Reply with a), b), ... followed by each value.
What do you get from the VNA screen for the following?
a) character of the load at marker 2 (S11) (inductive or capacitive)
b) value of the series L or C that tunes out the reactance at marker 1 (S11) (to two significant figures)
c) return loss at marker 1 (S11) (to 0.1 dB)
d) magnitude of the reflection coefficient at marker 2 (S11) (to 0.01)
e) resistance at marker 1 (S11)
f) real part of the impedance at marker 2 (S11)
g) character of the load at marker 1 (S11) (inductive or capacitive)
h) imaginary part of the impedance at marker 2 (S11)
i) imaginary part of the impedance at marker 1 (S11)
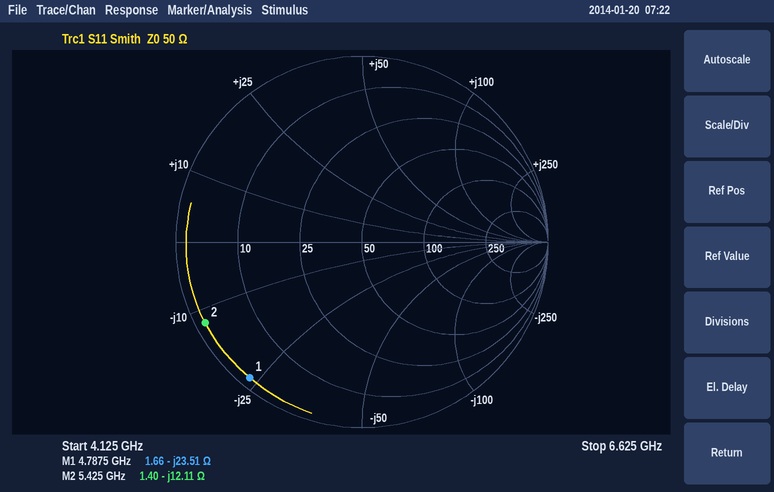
a) capacitive
b) 780 pH
c) 0.5 dB
d) 0.95
e) 1.66 Ω
f) 1.40 Ω
g) capacitive
h) -12.11 Ω
i) -23.51 Ω
